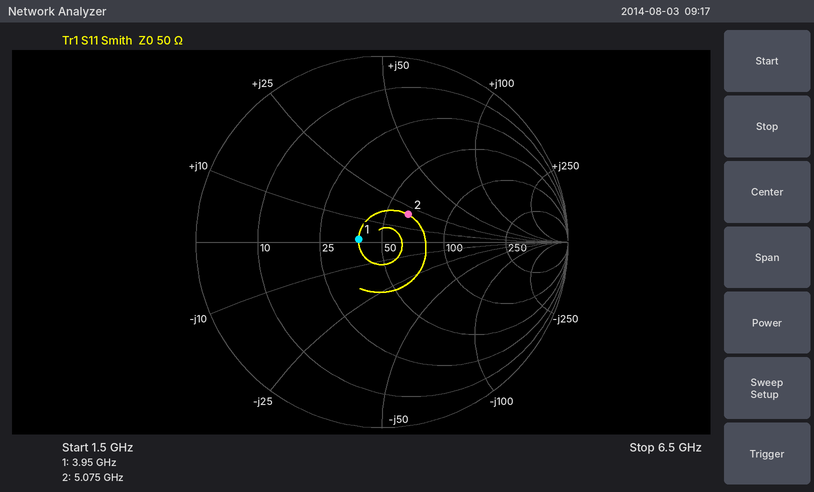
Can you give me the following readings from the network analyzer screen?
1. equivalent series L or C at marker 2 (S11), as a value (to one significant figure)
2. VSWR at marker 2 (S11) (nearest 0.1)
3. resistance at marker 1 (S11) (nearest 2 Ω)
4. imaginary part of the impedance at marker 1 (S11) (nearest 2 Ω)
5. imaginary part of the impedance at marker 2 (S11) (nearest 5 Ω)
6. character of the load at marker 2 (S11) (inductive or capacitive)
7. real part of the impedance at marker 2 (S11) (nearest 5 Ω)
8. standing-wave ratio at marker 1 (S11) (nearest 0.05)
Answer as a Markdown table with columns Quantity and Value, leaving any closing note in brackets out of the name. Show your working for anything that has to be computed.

| Quantity | Value |
|---|---|
| equivalent series L or C at marker 2 (S11), as a value | L = 20 Ω/(2π × 5.075 GHz) ≈ 627 pH, so 600 pH to one significant figure |
| VSWR at marker 2 (S11) | 1.5 |
| resistance at marker 1 (S11) | 38 Ω |
| imaginary part of the impedance at marker 1 (S11) | +2 Ω |
| imaginary part of the impedance at marker 2 (S11) | +20 Ω |
| character of the load at marker 2 (S11) | inductive |
| real part of the impedance at marker 2 (S11) | 65 Ω |
| standing-wave ratio at marker 1 (S11) | 1.30 |
